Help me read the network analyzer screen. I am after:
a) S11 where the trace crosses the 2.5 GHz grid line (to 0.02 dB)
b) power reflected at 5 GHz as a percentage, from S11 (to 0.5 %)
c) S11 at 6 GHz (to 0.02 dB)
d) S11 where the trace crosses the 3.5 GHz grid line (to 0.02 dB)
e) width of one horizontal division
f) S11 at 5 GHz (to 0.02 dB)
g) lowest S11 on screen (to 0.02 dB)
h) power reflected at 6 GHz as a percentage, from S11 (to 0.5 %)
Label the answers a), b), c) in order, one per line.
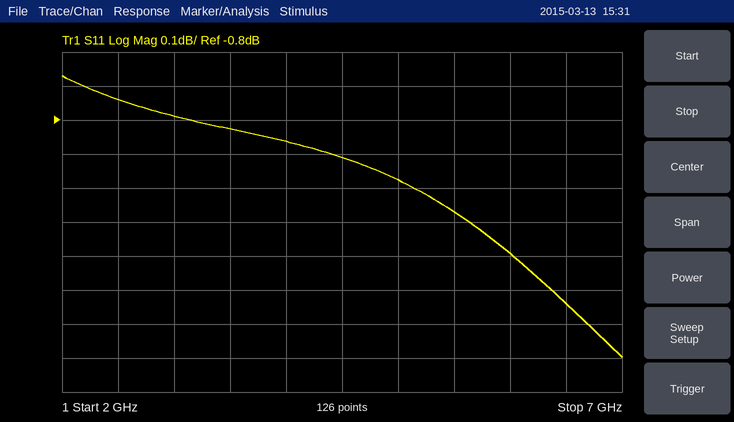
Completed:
a) -0.74 dB
b) 80.0 %
c) -1.20 dB
d) -0.82 dB
e) 500 MHz
f) -0.98 dB
g) -1.50 dB
h) 76.0 %
